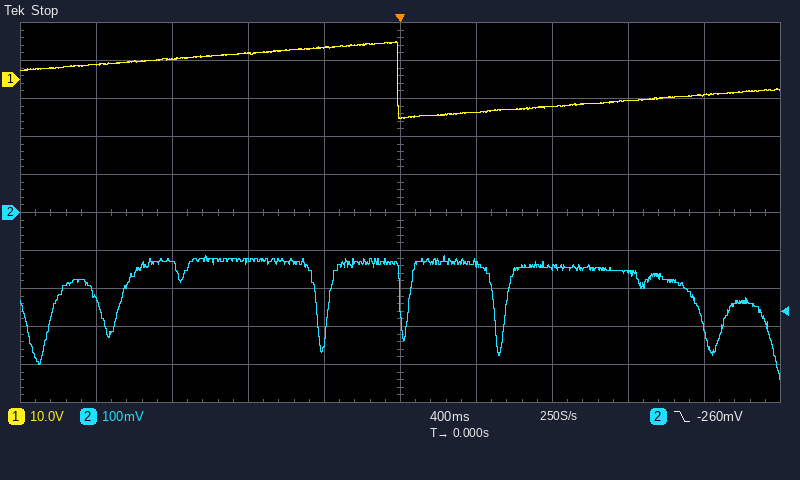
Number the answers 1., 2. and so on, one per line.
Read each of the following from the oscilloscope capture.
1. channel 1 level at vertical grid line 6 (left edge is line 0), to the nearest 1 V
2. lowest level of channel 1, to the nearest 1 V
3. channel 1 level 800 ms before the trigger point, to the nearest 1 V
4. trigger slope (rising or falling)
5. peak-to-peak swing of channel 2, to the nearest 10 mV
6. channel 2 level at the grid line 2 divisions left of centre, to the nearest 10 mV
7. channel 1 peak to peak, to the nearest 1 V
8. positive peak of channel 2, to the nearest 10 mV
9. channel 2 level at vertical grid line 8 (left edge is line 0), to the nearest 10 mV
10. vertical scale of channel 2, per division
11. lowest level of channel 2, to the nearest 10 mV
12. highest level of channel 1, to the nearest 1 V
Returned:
1. -9 V
2. -10 V
3. 7 V
4. falling
5. 330 mV
6. -130 mV
7. 20 V
8. -110 mV
9. -160 mV
10. 100 mV
11. -440 mV
12. 10 V
